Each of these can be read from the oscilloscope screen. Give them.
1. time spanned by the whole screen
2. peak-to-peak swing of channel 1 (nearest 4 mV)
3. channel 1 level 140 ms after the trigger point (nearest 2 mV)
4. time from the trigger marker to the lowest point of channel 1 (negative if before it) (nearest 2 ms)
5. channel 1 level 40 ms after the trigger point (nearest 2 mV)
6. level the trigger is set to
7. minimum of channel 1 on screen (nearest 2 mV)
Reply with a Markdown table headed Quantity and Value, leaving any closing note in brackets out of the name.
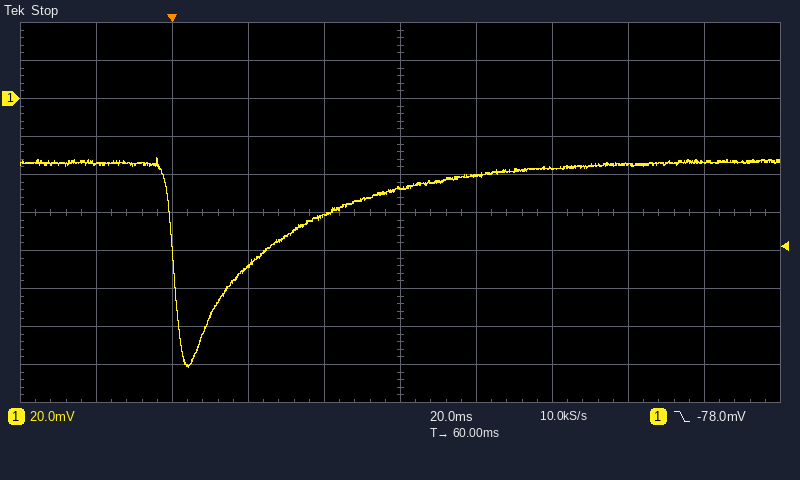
| Quantity | Value |
|---|---|
| time spanned by the whole screen | 200 ms |
| peak-to-peak swing of channel 1 | 112 mV |
| channel 1 level 140 ms after the trigger point | -34 mV |
| time from the trigger marker to the lowest point of channel 1 (negative if before it) | +4 ms |
| channel 1 level 40 ms after the trigger point | -62 mV |
| level the trigger is set to | -78.0 mV |
| minimum of channel 1 on screen | -142 mV |
